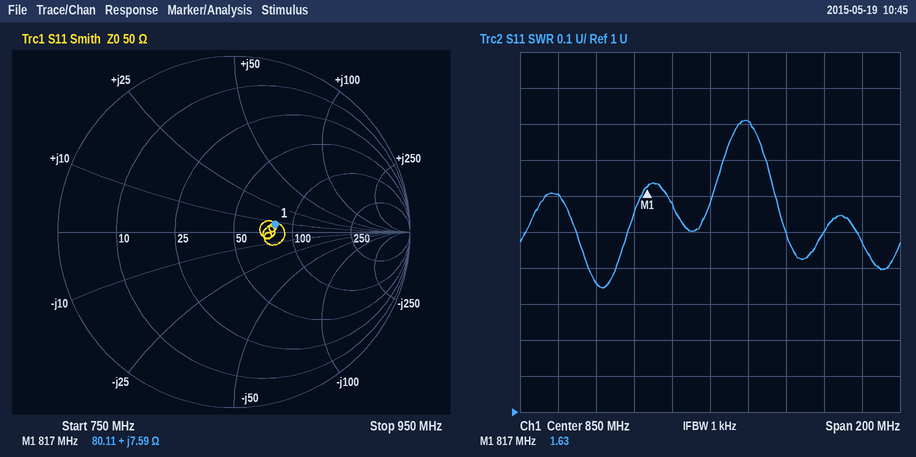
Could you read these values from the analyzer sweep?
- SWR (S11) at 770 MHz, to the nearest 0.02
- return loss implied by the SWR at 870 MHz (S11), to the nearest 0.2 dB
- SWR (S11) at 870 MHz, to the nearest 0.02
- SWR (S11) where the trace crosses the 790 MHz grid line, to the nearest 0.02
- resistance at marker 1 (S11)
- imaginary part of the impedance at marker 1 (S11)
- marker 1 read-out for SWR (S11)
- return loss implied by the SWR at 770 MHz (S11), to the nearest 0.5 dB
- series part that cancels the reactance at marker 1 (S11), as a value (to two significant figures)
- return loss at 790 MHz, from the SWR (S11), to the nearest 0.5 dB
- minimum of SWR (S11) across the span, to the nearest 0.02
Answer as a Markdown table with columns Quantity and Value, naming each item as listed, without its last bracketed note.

| Quantity | Value |
|---|---|
| SWR (S11) at 770 MHz, to the nearest 0.02 | 1.60 |
| return loss implied by the SWR at 870 MHz (S11), to the nearest 0.2 dB | 10.8 dB |
| SWR (S11) at 870 MHz, to the nearest 0.02 | 1.80 |
| SWR (S11) where the trace crosses the 790 MHz grid line, to the nearest 0.02 | 1.36 |
| resistance at marker 1 | 80.11 Ω |
| imaginary part of the impedance at marker 1 | +7.59 Ω |
| marker 1 read-out for SWR | 1.63 |
| return loss implied by the SWR at 770 MHz (S11), to the nearest 0.5 dB | 12.5 dB |
| series part that cancels the reactance at marker 1 (S11), as a value | 26 pF |
| return loss at 790 MHz, from the SWR (S11), to the nearest 0.5 dB | 16.5 dB |
| minimum of SWR (S11) across the span, to the nearest 0.02 | 1.34 |
